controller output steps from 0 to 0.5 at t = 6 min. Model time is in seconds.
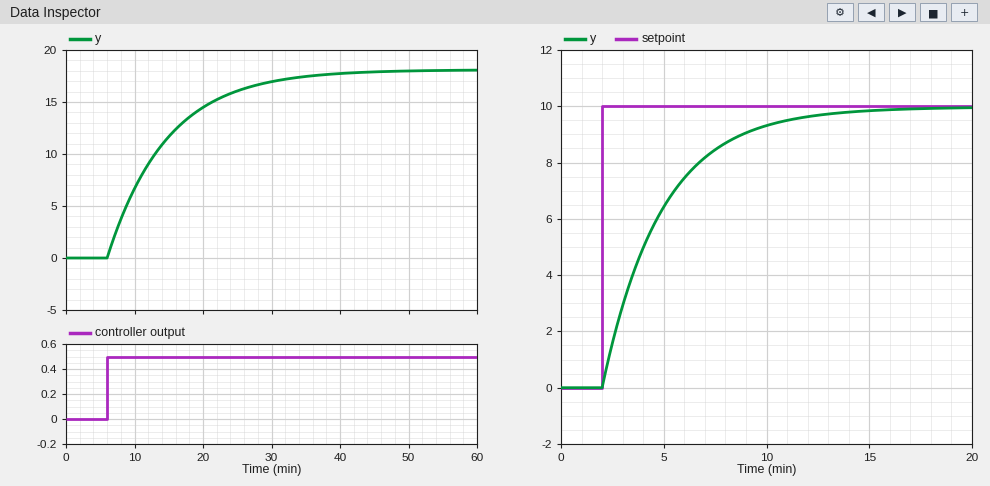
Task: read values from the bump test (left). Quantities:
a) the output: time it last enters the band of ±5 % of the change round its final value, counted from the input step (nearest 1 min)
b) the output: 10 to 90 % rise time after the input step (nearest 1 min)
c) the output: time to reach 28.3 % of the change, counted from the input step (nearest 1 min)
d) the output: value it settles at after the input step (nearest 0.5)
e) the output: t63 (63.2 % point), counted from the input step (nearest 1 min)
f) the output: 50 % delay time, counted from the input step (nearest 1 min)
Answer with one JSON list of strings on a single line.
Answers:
["26 min", "19 min", "3 min", "18.0", "9 min", "6 min"]
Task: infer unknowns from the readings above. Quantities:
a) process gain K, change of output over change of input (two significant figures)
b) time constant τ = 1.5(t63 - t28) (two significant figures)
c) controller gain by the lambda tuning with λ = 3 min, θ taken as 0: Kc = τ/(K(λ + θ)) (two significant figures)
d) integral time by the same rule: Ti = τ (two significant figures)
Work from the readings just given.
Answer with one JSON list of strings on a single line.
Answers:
["36", "9.0 min", "0.083", "9.0 min"]
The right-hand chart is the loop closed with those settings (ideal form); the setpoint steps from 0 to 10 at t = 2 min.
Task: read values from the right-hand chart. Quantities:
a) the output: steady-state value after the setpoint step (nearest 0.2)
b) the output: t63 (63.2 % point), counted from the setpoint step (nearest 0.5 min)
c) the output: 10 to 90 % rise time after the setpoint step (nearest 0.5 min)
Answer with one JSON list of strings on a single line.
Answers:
["10.0", "3.0 min", "6.5 min"]
